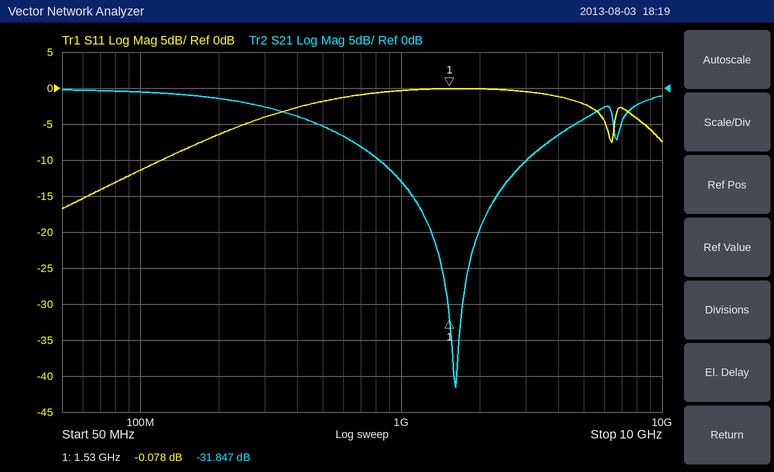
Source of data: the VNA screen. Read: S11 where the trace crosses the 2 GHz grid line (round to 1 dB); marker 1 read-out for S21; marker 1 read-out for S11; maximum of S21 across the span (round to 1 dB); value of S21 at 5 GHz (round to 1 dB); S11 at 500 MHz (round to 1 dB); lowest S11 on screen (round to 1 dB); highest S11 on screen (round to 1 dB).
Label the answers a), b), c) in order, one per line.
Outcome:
a) 0 dB
b) -31.847 dB
c) -0.078 dB
d) 0 dB
e) -4 dB
f) -2 dB
g) -17 dB
h) 0 dB
